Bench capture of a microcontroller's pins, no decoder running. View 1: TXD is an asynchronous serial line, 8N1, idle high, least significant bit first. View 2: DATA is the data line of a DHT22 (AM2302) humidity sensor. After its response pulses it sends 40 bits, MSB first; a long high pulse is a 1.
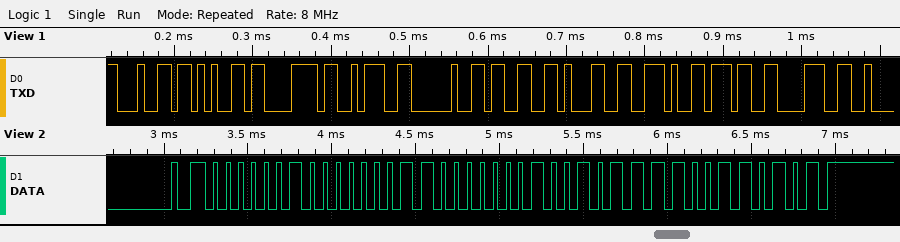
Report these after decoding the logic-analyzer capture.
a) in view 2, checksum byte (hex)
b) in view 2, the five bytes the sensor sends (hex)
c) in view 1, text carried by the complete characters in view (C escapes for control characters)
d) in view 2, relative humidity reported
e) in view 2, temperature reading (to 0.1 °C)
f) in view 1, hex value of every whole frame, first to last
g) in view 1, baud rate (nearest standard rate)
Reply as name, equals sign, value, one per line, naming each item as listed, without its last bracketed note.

in view 2, checksum byte = 0x35
in view 2, the five bytes the sensor sends = 02 03 01 2F 35
in view 1, text carried by the complete characters in view = "dex: 31.78"
in view 2, relative humidity reported = 51.5 %
in view 2, temperature reading = 30.3 °C
in view 1, hex value of every whole frame, first to last = 64 65 78 3A 20 33 31 2E 37 38
in view 1, baud rate = 115200 baud
